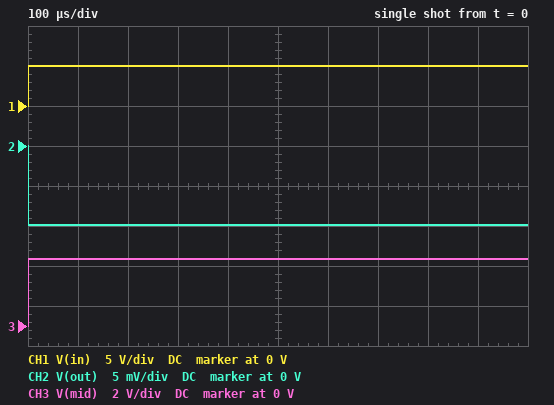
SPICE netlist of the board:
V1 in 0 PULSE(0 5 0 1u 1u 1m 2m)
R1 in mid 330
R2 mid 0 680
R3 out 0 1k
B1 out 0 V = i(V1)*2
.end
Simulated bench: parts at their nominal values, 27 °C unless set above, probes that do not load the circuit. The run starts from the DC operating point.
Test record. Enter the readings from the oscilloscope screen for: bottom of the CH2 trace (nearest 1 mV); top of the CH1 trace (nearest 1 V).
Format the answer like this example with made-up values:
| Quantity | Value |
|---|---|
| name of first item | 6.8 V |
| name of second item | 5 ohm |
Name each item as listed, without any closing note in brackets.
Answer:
| Quantity | Value |
|---|---|
| bottom of the CH2 trace | -10 mV |
| top of the CH1 trace | 5 V |
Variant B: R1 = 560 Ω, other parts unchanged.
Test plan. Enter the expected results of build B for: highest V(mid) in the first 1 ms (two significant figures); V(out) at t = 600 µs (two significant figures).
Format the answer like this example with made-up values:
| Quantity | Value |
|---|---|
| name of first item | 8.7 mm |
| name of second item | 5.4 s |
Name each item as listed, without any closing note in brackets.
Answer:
| Quantity | Value |
|---|---|
| highest V(mid) in the first 1 ms | 2.7 V |
| V(out) at t = 600 µs | -8.1 mV |
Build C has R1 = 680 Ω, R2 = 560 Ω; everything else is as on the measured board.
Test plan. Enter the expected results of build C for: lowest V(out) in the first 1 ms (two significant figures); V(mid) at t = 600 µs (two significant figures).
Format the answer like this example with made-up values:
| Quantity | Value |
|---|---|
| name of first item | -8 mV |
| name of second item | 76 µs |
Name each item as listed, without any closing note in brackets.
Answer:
| Quantity | Value |
|---|---|
| lowest V(out) in the first 1 ms | -8.1 mV |
| V(mid) at t = 600 µs | 2.3 V |
